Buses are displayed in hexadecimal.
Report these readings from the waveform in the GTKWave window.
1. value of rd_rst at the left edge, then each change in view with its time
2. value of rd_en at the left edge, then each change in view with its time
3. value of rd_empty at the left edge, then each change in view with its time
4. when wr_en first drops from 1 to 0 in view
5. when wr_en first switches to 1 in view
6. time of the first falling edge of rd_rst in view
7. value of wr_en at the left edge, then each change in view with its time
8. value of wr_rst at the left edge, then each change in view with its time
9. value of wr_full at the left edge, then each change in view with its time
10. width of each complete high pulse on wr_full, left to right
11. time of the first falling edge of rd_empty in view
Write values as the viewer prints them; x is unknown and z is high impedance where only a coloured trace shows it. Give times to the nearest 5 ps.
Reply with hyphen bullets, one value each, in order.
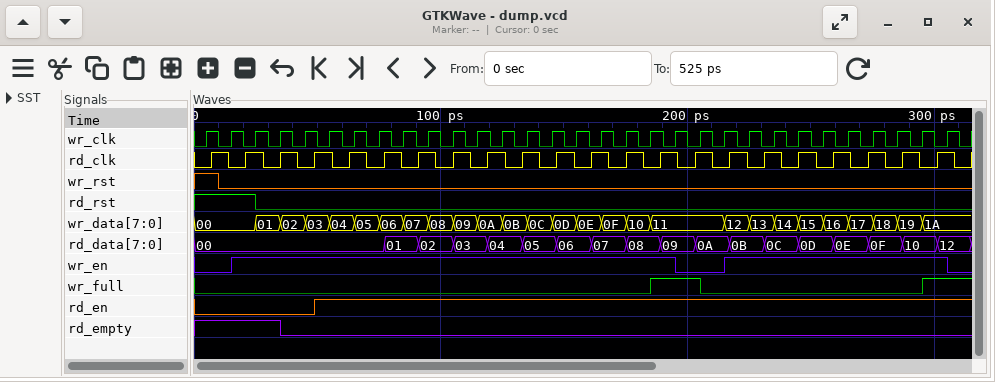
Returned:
- 1, 0 at 25 ps
- 0, 1 at 50 ps
- 1, 0 at 35 ps
- 195 ps
- 15 ps
- 25 ps
- 0, 1 at 15 ps, 0 at 195 ps, 1 at 215 ps, 0 at 305 ps
- 1, 0 at 10 ps
- 0, 1 at 185 ps, 0 at 205 ps, 1 at 295 ps
- 20 ps
- 35 ps
